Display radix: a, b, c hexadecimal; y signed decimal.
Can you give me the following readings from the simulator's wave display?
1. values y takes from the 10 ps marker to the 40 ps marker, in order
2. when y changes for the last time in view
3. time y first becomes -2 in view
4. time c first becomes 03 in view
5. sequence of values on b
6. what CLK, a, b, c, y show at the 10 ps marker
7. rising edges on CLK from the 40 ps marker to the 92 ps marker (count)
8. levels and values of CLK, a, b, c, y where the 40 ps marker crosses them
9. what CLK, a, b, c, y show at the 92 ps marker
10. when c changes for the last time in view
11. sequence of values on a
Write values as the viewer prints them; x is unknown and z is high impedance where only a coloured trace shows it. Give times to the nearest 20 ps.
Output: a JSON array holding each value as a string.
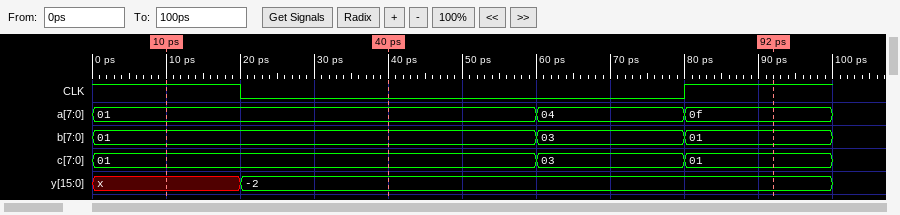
["x, -2", "20 ps", "20 ps", "60 ps", "01, 03, 01", "CLK=1, a=01, b=01, c=01, y=x", "1", "CLK=0, a=01, b=01, c=01, y=-2", "CLK=1, a=0f, b=01, c=01, y=-2", "80 ps", "01, 04, 0f"]
